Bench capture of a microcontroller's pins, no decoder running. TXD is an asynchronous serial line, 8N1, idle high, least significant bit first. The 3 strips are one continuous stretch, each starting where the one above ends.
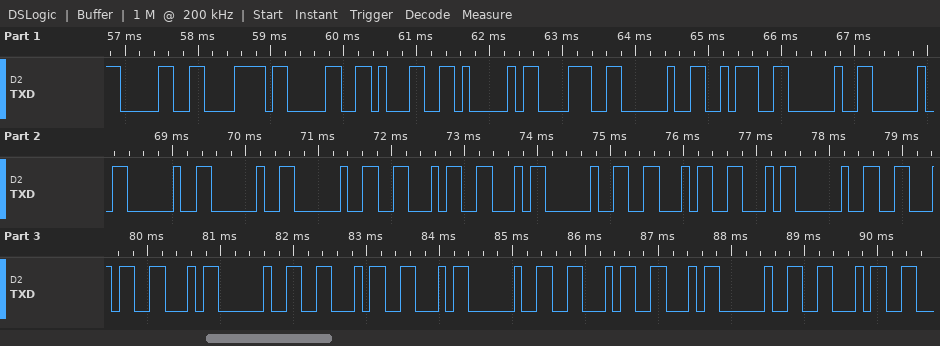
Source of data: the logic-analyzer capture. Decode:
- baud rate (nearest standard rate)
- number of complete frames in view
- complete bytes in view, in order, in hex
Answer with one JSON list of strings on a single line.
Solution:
["9600 baud", "29", "0x30 0x78 0x30 0x31 0x41 0x38 0x20 0x3A 0x20 0x20 0x20 0x20 0x20 0x46 0x46 0x20 0x46 0x46 0x20 0x46 0x46 0x20 0x46 0x46 0x20 0x46 0x46 0x20 0x46"]
